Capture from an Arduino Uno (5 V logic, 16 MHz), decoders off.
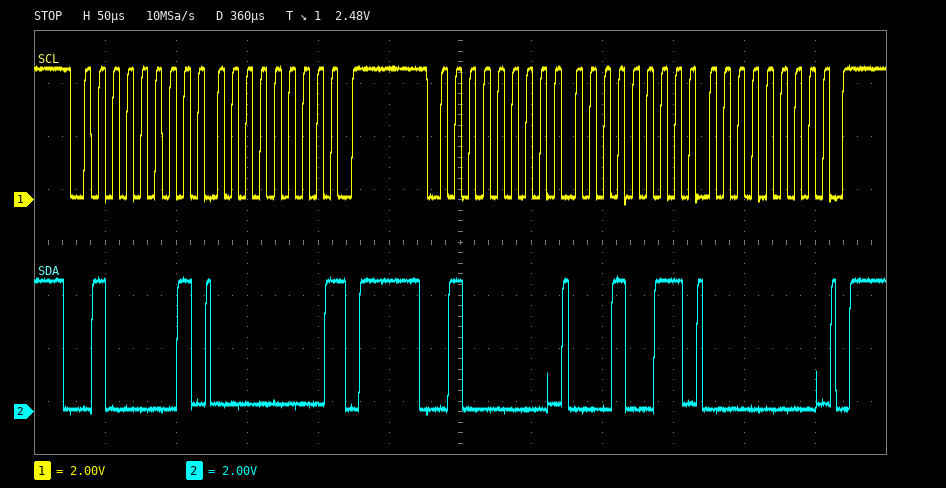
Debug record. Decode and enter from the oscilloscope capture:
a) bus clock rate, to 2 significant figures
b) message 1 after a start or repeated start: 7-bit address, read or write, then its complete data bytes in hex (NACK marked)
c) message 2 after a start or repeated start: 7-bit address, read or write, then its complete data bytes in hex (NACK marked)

100 kHz
0x20 read: 00 NACK
0x20 write: 13 00
